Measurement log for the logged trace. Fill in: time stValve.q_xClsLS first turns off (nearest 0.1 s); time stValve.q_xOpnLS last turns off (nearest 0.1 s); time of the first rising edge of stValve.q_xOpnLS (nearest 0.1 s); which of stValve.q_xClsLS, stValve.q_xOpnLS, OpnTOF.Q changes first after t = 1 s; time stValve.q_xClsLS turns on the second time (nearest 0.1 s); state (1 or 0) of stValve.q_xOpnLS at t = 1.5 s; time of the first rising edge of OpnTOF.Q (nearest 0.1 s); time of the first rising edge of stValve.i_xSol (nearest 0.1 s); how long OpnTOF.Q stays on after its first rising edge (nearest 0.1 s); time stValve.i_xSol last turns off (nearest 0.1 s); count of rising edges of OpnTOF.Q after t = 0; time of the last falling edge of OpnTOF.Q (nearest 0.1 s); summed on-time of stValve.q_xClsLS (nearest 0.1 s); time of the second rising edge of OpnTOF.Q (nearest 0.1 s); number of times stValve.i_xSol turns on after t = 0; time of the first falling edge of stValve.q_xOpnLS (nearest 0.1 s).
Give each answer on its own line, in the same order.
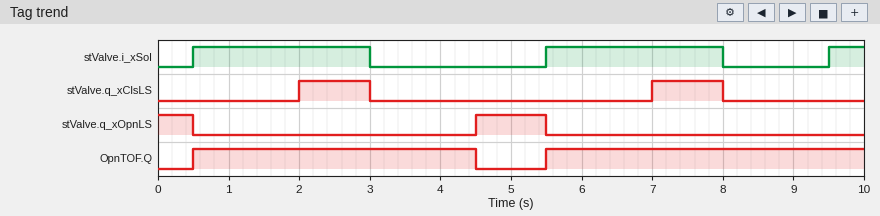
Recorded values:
3.0 s
5.5 s
4.5 s
stValve.q_xClsLS
7.0 s
0
0.5 s
0.5 s
4.0 s
8.0 s
2
4.5 s
2.0 s
5.5 s
3
0.5 s
